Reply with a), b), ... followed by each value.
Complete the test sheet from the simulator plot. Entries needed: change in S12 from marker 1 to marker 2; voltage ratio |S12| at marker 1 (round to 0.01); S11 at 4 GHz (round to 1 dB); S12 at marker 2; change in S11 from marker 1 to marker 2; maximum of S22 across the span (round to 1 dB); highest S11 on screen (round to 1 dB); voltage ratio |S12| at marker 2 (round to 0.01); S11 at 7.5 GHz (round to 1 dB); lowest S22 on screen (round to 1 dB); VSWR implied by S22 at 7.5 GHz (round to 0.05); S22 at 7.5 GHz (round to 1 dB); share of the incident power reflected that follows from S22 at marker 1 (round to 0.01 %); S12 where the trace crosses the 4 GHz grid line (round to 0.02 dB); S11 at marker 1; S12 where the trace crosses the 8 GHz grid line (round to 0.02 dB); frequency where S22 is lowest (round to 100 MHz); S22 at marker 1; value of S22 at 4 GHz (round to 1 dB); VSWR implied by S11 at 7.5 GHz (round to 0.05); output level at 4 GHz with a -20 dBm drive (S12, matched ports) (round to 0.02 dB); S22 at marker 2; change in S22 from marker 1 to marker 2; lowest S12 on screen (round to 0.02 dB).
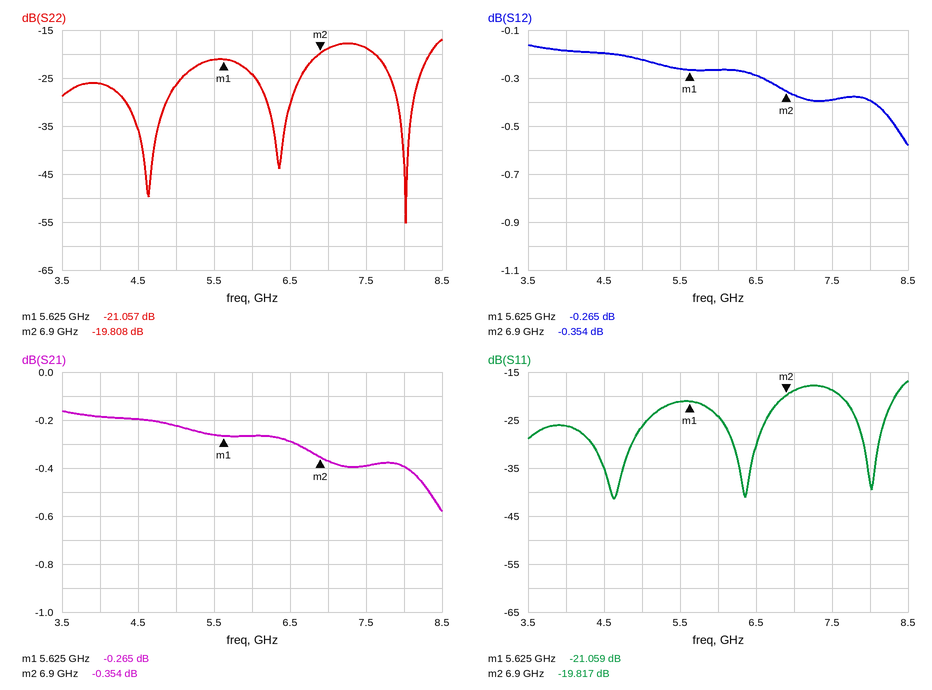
a) -0.089 dB
b) 0.97
c) -26 dB
d) -0.354 dB
e) 1.242 dB
f) -17 dB
g) -17 dB
h) 0.96
i) -19 dB
j) -55 dB
k) 1.25
l) -19 dB
m) 0.78 %
n) -0.18 dB
o) -21.059 dB
p) -0.40 dB
q) 8.0 GHz
r) -21.057 dB
s) -26 dB
t) 1.25
u) -20.18 dBm
v) -19.808 dB
w) 1.249 dB
x) -0.58 dB
